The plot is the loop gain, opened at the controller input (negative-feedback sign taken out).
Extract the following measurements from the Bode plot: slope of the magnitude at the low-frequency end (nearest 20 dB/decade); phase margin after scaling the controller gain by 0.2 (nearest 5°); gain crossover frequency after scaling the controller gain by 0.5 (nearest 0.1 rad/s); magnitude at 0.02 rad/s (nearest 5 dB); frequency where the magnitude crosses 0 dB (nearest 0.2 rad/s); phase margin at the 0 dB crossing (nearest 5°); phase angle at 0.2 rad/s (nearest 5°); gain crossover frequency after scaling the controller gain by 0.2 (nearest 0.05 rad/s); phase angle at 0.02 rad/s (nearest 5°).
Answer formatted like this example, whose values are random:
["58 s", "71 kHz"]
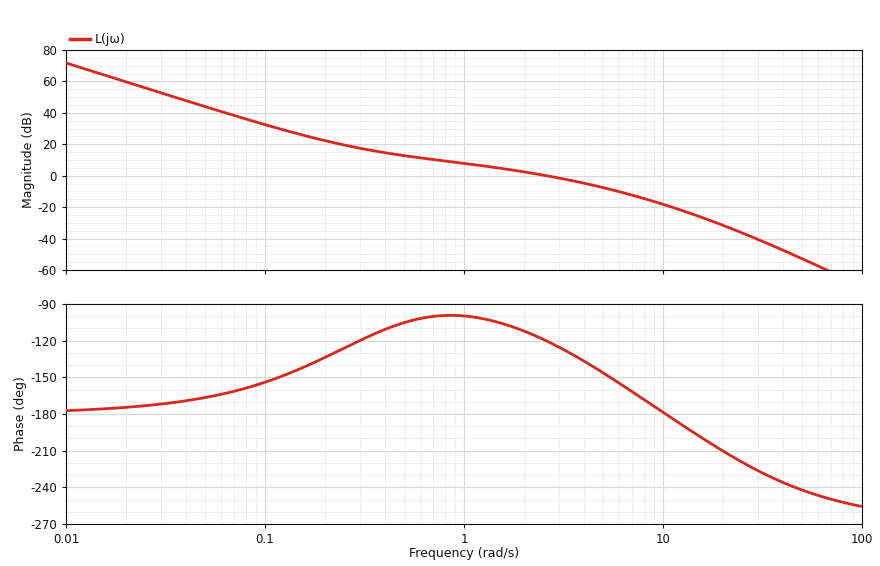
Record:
["-40 dB/decade", "70°", "1.3 rad/s", "60 dB", "2.6 rad/s", "60°", "-135°", "0.45 rad/s", "-175°"]
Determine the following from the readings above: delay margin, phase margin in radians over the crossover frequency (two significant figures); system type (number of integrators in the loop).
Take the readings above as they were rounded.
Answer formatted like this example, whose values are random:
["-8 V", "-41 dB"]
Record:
["0.40 s", "2"]
